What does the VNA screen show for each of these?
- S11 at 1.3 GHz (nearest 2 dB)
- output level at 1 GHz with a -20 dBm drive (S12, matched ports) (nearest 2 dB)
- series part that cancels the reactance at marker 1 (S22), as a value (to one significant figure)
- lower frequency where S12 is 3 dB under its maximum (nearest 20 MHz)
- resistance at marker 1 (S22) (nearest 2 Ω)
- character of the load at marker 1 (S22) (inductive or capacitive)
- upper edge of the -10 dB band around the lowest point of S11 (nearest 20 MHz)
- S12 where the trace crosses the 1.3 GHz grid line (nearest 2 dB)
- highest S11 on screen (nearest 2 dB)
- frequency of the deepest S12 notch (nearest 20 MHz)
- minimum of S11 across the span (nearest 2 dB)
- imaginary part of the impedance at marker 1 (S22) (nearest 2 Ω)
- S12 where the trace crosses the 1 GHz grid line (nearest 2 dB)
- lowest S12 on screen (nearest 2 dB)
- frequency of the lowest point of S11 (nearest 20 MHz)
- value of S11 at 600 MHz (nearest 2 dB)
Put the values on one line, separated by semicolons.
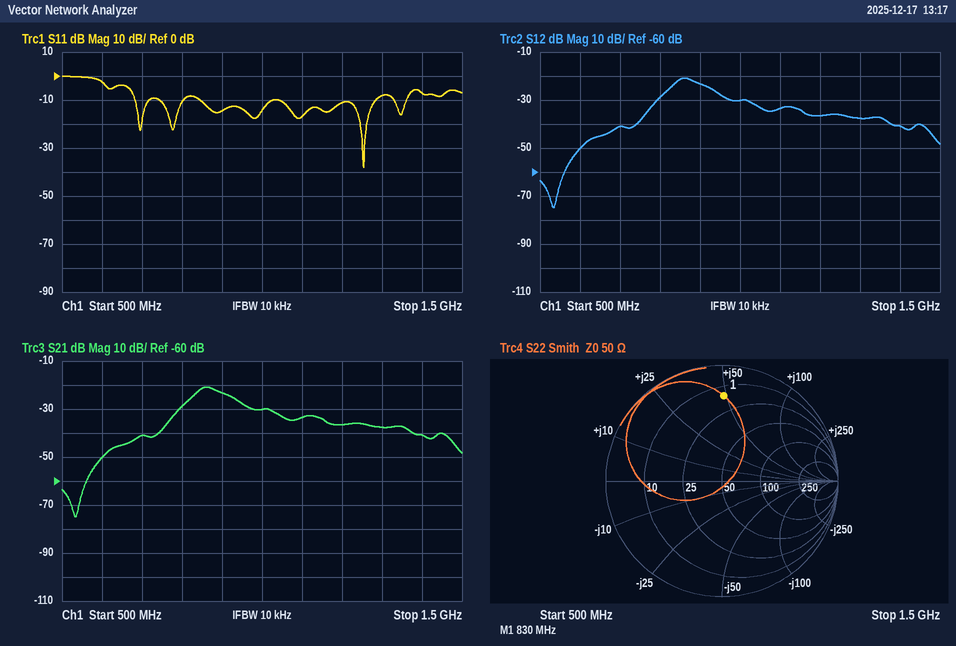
-8 dB; -50 dBm; 4 pF; 840 MHz; 16 Ω; inductive; 1.28 GHz; -38 dB; 0 dB; 540 MHz; -38 dB; +48 Ω; -30 dB; -74 dB; 1.26 GHz; -2 dB
